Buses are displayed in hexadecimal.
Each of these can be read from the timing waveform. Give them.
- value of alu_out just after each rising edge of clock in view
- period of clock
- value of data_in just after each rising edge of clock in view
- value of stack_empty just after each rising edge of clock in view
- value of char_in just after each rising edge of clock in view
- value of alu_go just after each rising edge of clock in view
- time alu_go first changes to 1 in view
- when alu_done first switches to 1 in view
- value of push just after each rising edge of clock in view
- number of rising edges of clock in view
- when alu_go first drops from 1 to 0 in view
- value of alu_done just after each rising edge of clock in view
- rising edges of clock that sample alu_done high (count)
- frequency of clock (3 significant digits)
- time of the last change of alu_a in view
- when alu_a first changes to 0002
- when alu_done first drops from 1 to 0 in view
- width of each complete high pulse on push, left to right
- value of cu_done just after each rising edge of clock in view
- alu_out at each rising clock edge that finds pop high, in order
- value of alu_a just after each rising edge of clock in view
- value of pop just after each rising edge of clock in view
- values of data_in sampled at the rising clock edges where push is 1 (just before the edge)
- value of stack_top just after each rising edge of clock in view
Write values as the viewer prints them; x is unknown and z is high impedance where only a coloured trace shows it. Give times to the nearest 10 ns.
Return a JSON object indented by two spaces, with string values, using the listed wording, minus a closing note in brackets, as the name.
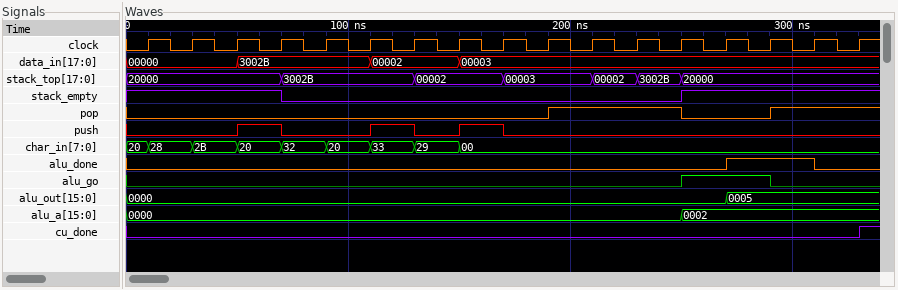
{
  "value of alu_out just after each rising edge of clock in view": "0000, 0000, 0000, 0000, 0000, 0000, 0000, 0000, 0000, 0000, 0000, 0000, 0000, 0005, 0005, 0005, 0005",
  "period of clock": "20 ns",
  "value of data_in just after each rising edge of clock in view": "00000, 00000, 3002B, 3002B, 3002B, 00002, 00002, 00003, 00003, 00003, 00003, 00003, 00003, 00003, 00003, 00003, 00003",
  "value of stack_empty just after each rising edge of clock in view": "1 1 1 0 0 0 0 0 0 0 0 0 1 1 1 1 1",
  "value of char_in just after each rising edge of clock in view": "28, 2B, 20, 32, 20, 33, 29, 00, 00, 00, 00, 00, 00, 00, 00, 00, 00",
  "value of alu_go just after each rising edge of clock in view": "0 0 0 0 0 0 0 0 0 0 0 0 1 1 0 0 0",
  "time alu_go first changes to 1 in view": "250 ns",
  "when alu_done first switches to 1 in view": "270 ns",
  "value of push just after each rising edge of clock in view": "0 0 1 0 0 1 0 1 0 0 0 0 0 0 0 0 0",
  "number of rising edges of clock in view": "17",
  "when alu_go first drops from 1 to 0 in view": "290 ns",
  "value of alu_done just after each rising edge of clock in view": "0 0 0 0 0 0 0 0 0 0 0 0 0 1 1 0 0",
  "rising edges of clock that sample alu_done high": "2",
  "frequency of clock": "50.0 MHz",
  "time of the last change of alu_a in view": "250 ns",
  "when alu_a first changes to 0002": "250 ns",
  "when alu_done first drops from 1 to 0 in view": "310 ns",
  "width of each complete high pulse on push, left to right": "20 ns, 20 ns, 20 ns",
  "value of cu_done just after each rising edge of clock in view": "0 0 0 0 0 0 0 0 0 0 0 0 0 0 0 0 1",
  "alu_out at each rising clock edge that finds pop high, in order": "0000, 0000, 0000, 0005, 0005",
  "value of alu_a just after each rising edge of clock in view": "0000, 0000, 0000, 0000, 0000, 0000, 0000, 0000, 0000, 0000, 0000, 0000, 0002, 0002, 0002, 0002, 0002",
  "value of pop just after each rising edge of clock in view": "0 0 0 0 0 0 0 0 0 1 1 1 0 0 1 1 1",
  "values of data_in sampled at the rising clock edges where push is 1": "3002B, 00002, 00003",
  "value of stack_top just after each rising edge of clock in view": "20000, 20000, 20000, 3002B, 3002B, 3002B, 00002, 00002, 00003, 00003, 00002, 3002B, 20000, 20000, 20000, 20000, 20000"
}
